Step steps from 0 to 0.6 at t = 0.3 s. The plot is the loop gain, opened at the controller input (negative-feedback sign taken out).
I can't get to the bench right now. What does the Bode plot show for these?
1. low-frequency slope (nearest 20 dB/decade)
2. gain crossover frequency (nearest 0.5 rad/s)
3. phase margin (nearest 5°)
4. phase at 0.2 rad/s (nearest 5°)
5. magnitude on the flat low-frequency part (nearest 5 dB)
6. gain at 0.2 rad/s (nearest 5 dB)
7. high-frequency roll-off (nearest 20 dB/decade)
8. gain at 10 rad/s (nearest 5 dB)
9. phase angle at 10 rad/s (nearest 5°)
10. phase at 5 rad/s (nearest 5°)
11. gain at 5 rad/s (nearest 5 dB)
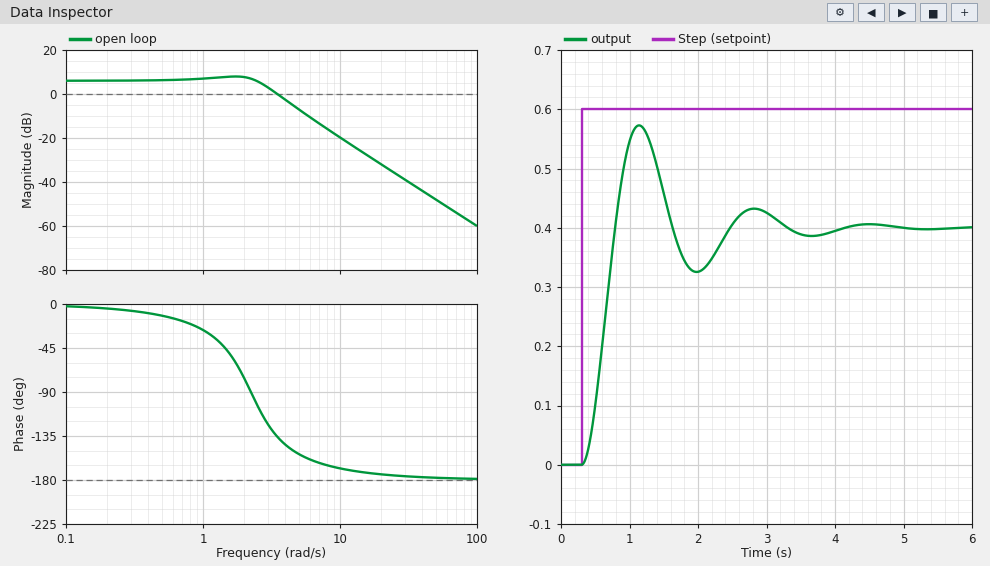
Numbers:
0 dB/decade
3.5 rad/s
45°
-5°
5 dB
5 dB
-40 dB/decade
-20 dB
-170°
-155°
-5 dB
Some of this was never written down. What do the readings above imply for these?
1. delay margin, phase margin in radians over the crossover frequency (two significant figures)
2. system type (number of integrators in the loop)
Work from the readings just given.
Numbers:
0.22 s
0
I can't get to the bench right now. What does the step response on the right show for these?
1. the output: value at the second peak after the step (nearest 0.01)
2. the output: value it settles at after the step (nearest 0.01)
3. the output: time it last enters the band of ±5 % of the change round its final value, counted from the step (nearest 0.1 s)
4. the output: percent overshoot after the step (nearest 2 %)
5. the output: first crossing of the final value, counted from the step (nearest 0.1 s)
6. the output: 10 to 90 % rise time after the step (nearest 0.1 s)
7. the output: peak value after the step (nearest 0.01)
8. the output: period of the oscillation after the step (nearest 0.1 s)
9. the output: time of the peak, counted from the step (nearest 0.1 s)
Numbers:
0.43
0.40
2.8 s
44 %
0.5 s
0.3 s
0.57
1.7 s
0.8 s
